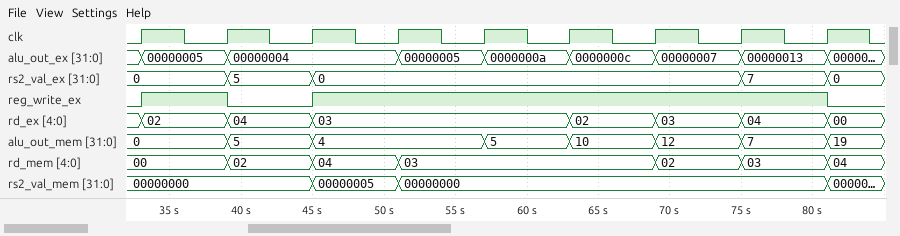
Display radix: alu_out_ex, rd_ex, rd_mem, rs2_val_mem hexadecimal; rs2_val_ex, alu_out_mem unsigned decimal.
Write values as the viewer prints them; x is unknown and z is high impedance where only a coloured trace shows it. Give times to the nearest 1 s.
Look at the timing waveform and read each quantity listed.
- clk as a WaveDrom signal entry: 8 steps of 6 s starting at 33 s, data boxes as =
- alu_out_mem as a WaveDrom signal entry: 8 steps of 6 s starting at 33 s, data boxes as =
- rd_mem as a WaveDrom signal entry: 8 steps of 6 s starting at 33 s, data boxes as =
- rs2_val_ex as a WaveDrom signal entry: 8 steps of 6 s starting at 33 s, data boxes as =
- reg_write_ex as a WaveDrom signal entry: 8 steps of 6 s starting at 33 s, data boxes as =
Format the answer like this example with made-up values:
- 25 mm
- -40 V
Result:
- {name: 'clk', wave: 'p.......'}
- {name: 'alu_out_mem', wave: '===.====', data: '0 5 4 5 10 12 7'}
- {name: 'rd_mem', wave: '====..==', data: '00 02 04 03 02 03'}
- {name: 'rs2_val_ex', wave: '===....=', data: '0 5 0 7'}
- {name: 'reg_write_ex', wave: '101.....'}
